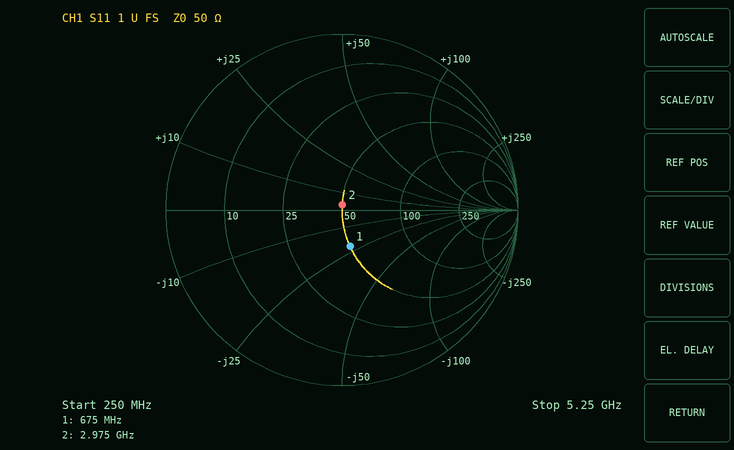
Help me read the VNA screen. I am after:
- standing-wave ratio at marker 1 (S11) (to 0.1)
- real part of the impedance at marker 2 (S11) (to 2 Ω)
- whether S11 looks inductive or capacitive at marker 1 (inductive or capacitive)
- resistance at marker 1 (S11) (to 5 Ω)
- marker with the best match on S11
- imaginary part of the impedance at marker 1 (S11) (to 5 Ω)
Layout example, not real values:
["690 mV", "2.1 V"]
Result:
["1.5", "50 Ω", "capacitive", "50 Ω", "marker 2", "-20 Ω"]
